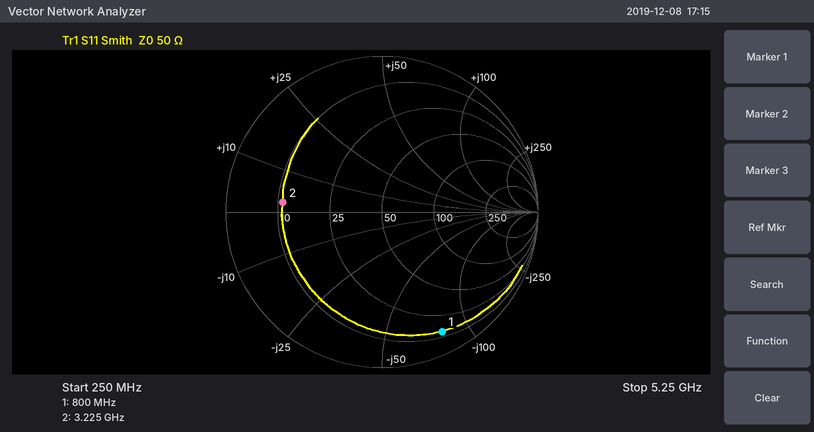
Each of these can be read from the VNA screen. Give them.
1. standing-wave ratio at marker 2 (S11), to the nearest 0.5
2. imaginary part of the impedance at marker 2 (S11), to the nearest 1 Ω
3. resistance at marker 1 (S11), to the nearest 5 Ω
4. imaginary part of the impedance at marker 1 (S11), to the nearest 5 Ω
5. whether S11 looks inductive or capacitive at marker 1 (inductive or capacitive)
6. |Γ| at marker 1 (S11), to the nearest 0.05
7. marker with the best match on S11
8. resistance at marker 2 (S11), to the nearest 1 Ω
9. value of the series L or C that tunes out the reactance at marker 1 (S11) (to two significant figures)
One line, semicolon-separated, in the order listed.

4.5; +2 Ω; 15 Ω; -80 Ω; capacitive; 0.85; marker 2; 11 Ω; 16 nH
